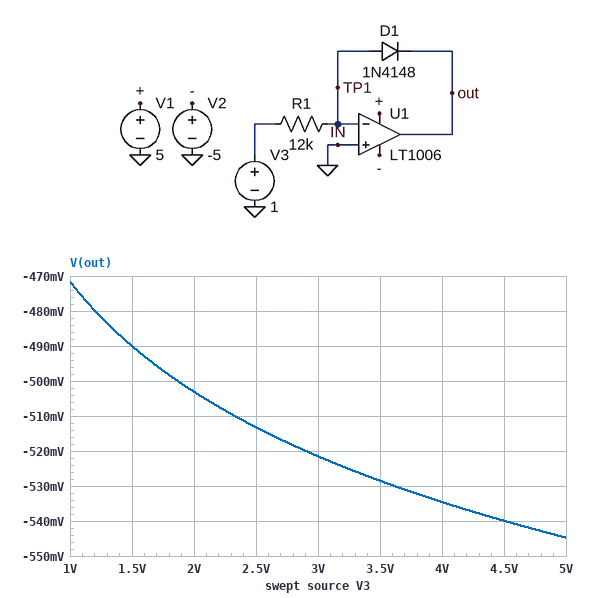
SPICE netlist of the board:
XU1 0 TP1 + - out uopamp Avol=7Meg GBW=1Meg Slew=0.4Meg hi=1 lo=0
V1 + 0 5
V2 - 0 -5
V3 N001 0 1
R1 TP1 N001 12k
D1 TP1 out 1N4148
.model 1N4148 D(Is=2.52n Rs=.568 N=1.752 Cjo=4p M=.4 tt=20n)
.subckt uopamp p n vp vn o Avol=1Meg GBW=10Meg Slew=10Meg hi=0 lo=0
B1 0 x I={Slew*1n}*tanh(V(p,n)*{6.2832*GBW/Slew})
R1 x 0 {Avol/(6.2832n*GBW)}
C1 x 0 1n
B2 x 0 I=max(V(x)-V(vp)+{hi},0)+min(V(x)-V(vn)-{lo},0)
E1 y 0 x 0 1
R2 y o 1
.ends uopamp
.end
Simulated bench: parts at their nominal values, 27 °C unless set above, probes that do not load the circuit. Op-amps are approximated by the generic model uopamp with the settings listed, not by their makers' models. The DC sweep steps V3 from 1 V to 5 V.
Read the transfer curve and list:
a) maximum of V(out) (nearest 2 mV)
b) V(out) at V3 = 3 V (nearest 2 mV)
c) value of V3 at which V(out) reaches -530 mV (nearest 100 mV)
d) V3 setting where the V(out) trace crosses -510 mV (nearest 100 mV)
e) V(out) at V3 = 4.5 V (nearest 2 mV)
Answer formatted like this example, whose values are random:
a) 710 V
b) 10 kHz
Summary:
a) -472 mV
b) -522 mV
c) 3.6 V
d) 2.3 V
e) -540 mV
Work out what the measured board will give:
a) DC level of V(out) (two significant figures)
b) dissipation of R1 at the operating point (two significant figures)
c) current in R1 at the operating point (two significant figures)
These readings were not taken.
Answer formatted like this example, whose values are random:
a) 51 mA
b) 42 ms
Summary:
a) -470 mV
b) 83 µW
c) 83 µA
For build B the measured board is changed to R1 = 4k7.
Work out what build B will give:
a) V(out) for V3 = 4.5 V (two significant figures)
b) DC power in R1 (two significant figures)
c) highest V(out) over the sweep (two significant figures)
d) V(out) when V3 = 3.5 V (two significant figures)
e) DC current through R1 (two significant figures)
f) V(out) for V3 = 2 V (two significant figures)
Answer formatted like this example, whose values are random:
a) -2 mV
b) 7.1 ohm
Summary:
a) -580 mV
b) 210 µW
c) -510 mV
d) -570 mV
e) 210 µA
f) -550 mV
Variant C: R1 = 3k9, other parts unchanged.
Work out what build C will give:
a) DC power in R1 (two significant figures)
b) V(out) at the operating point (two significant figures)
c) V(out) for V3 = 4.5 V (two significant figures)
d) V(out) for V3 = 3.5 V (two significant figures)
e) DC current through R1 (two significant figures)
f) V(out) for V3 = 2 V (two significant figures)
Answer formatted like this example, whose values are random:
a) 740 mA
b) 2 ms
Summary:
a) 260 µW
b) -520 mV
c) -590 mV
d) -580 mV
e) 260 µA
f) -550 mV
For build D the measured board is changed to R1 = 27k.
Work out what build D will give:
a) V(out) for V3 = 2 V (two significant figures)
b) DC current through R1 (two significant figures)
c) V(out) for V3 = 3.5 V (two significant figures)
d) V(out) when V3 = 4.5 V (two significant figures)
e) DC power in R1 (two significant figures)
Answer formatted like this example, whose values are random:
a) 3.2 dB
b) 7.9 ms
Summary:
a) -470 mV
b) 37 µA
c) -490 mV
d) -500 mV
e) 37 µW
